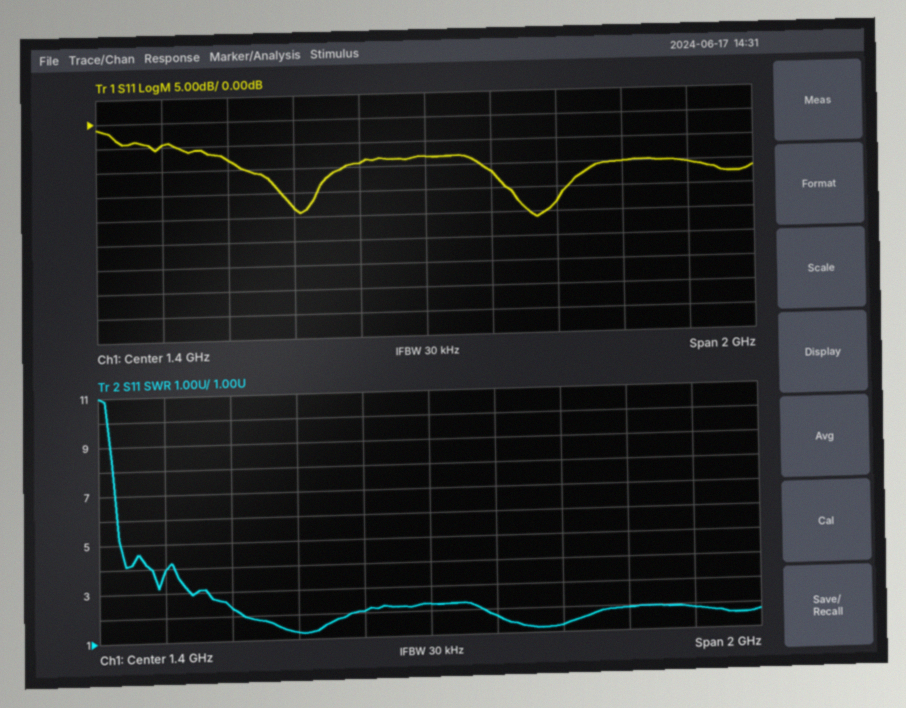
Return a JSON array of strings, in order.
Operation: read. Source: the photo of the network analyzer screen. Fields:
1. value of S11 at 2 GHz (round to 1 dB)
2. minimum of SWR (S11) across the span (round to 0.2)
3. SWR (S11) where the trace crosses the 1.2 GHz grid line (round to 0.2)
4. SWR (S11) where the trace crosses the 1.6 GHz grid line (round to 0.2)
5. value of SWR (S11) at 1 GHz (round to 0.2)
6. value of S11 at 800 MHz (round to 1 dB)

["-10 dB", "1.2", "2.0", "1.8", "1.2", "-8 dB"]
